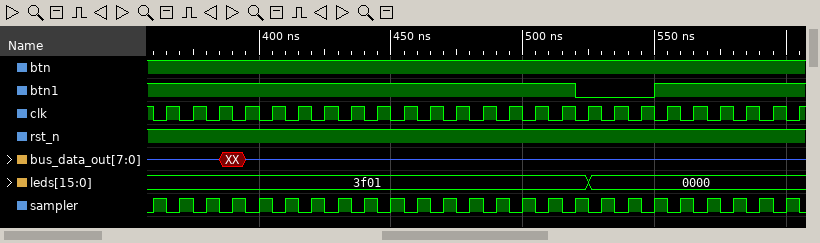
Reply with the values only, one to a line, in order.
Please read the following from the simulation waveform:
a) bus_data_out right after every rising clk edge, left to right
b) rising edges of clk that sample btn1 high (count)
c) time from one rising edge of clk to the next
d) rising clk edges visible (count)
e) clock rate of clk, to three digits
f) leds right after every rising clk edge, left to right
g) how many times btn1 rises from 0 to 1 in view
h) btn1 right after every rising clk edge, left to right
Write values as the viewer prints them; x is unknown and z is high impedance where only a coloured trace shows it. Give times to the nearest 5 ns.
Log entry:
z, z, XX, z, z, z, z, z, z, z, z, z, z, z, z, z, z, z, z, z, z, z, z, z, z
22
10 ns
25
100 MHz
3f01, 3f01, 3f01, 3f01, 3f01, 3f01, 3f01, 3f01, 3f01, 3f01, 3f01, 3f01, 3f01, 3f01, 3f01, 3f01, 0000, 0000, 0000, 0000, 0000, 0000, 0000, 0000, 0000
1
1 1 1 1 1 1 1 1 1 1 1 1 1 1 1 1 0 0 0 1 1 1 1 1 1
